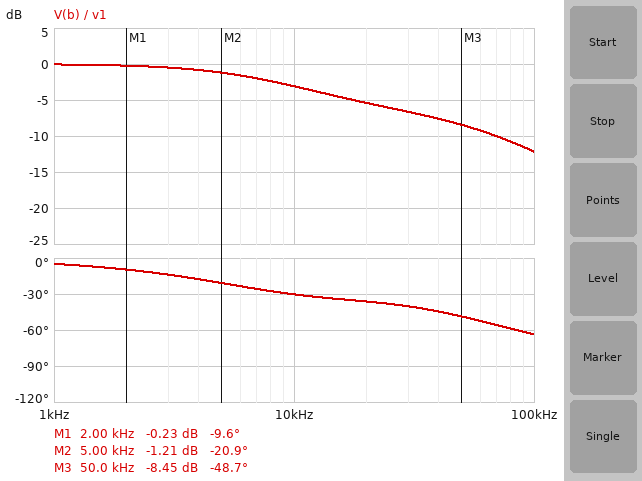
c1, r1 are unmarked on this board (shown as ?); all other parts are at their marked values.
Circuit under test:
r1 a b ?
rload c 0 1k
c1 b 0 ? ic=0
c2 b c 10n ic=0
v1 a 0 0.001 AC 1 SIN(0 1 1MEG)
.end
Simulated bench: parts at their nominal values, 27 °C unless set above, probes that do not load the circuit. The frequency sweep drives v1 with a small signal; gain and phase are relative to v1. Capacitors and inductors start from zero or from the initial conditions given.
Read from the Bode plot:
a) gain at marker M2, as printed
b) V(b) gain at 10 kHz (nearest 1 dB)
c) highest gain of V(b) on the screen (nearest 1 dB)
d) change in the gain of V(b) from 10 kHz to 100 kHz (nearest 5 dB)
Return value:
-1.21 dB
-3 dB
0 dB
-10 dB
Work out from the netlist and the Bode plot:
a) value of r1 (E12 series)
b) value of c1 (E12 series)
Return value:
820 Ω
6.8 nF
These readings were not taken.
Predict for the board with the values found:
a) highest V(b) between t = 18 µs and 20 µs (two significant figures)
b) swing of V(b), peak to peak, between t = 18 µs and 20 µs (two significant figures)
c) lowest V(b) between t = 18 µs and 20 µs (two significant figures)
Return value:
30 mV
57 mV
-27 mV
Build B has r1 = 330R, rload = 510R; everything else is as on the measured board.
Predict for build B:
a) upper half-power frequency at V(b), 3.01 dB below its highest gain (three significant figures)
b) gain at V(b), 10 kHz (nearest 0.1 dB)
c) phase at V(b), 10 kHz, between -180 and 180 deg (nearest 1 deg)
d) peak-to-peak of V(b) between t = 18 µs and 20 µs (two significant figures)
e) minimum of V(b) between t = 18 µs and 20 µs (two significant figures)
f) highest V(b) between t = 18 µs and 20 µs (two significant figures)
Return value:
24.7 kHz
-0.9 dB
-17 deg
140 mV
-69 mV
72 mV
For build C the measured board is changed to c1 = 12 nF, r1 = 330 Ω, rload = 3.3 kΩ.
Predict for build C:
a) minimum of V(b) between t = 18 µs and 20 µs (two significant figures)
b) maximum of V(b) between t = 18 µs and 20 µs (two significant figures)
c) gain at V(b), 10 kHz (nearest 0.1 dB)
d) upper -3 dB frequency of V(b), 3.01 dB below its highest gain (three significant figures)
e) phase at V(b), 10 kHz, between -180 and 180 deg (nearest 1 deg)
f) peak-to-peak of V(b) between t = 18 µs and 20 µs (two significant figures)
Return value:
-40 mV
41 mV
-1.0 dB
35.3 kHz
-15 deg
80 mV
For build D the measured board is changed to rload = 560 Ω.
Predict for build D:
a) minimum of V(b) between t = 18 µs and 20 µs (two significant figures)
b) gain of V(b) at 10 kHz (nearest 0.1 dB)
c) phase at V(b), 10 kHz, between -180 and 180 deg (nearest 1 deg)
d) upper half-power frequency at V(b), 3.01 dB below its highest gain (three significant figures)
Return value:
-26 mV
-3.0 dB
-35 deg
9.98 kHz
